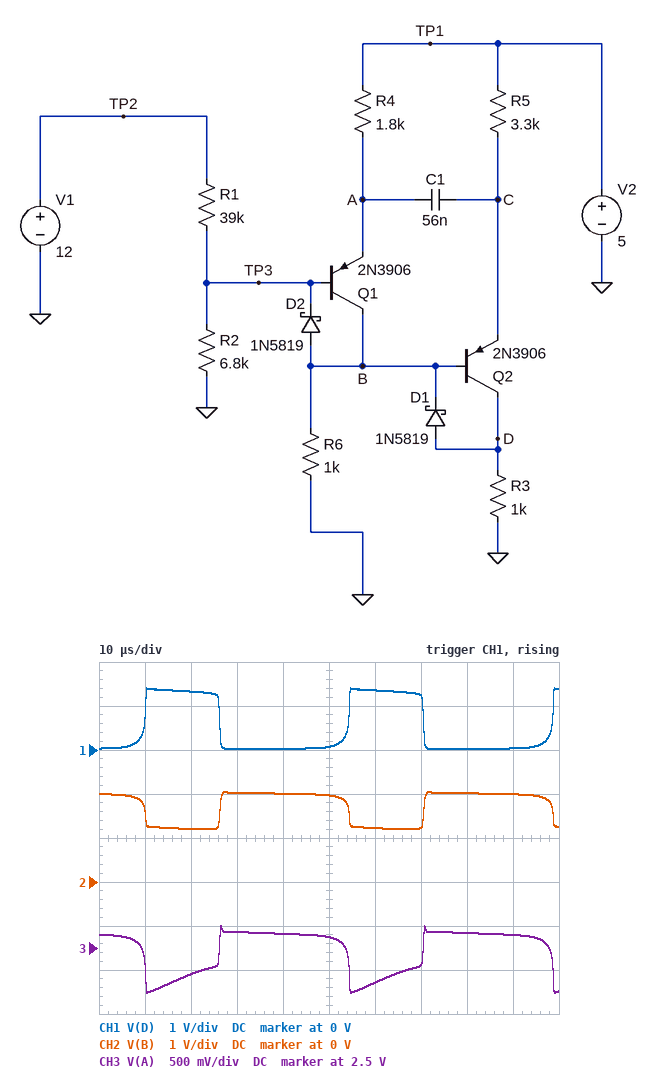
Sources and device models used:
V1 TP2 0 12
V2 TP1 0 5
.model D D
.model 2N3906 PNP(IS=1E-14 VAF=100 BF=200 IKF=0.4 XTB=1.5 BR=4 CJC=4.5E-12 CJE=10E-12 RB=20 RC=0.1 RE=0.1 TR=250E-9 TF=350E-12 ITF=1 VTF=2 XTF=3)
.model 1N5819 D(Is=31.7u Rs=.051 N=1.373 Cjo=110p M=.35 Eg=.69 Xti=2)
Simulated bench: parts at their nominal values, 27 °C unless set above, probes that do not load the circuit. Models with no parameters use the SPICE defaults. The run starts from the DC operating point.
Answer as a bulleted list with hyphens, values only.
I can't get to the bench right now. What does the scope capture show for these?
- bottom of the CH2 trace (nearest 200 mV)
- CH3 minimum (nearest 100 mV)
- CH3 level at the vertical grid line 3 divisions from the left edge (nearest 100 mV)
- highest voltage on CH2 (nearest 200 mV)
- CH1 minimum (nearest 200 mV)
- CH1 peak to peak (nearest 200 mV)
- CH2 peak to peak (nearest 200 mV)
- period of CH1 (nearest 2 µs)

- 1.2 V
- 2.0 V
- 2.7 V
- 2.0 V
- 0 V
- 1.4 V
- 800 mV
- 44 µs
